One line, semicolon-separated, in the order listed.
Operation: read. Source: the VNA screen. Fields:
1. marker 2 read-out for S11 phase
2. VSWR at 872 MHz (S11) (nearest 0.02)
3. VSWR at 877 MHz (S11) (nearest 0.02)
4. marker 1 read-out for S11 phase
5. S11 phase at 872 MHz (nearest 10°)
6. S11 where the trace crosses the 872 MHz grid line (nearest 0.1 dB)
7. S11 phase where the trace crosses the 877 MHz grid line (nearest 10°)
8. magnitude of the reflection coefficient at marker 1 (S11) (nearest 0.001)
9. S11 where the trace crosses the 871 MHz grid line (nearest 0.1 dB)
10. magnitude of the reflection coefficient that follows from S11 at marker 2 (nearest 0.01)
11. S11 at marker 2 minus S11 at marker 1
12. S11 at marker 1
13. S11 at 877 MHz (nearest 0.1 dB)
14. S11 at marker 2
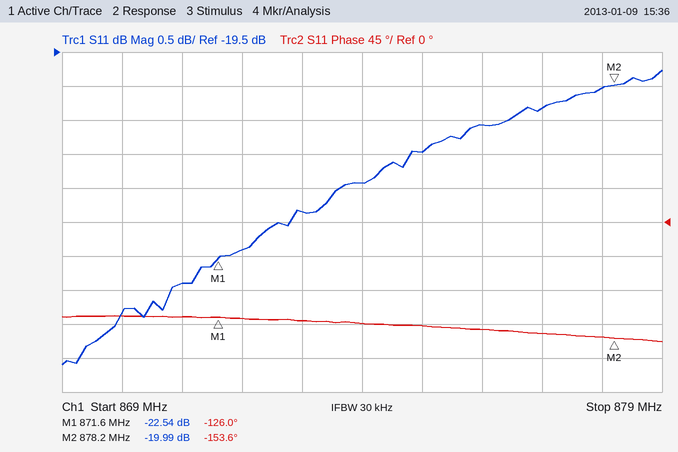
-153.6°; 1.16; 1.22; -126.0°; -130°; -22.4 dB; -150°; 0.075; -22.9 dB; 0.10; 2.55 dB; -22.54 dB; -20.3 dB; -19.99 dB
